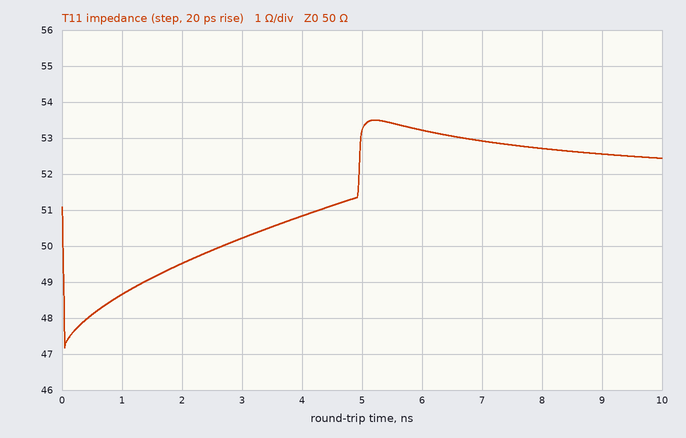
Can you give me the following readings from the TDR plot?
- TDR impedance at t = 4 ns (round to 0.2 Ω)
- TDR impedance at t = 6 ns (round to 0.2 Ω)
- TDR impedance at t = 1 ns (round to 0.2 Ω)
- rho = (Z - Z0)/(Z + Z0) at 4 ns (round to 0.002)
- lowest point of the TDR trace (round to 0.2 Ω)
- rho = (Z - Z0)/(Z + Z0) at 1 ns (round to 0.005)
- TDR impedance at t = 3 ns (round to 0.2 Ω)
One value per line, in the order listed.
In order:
50.8 Ω
53.2 Ω
48.6 Ω
+0.008
47.2 Ω
-0.015
50.2 Ω
